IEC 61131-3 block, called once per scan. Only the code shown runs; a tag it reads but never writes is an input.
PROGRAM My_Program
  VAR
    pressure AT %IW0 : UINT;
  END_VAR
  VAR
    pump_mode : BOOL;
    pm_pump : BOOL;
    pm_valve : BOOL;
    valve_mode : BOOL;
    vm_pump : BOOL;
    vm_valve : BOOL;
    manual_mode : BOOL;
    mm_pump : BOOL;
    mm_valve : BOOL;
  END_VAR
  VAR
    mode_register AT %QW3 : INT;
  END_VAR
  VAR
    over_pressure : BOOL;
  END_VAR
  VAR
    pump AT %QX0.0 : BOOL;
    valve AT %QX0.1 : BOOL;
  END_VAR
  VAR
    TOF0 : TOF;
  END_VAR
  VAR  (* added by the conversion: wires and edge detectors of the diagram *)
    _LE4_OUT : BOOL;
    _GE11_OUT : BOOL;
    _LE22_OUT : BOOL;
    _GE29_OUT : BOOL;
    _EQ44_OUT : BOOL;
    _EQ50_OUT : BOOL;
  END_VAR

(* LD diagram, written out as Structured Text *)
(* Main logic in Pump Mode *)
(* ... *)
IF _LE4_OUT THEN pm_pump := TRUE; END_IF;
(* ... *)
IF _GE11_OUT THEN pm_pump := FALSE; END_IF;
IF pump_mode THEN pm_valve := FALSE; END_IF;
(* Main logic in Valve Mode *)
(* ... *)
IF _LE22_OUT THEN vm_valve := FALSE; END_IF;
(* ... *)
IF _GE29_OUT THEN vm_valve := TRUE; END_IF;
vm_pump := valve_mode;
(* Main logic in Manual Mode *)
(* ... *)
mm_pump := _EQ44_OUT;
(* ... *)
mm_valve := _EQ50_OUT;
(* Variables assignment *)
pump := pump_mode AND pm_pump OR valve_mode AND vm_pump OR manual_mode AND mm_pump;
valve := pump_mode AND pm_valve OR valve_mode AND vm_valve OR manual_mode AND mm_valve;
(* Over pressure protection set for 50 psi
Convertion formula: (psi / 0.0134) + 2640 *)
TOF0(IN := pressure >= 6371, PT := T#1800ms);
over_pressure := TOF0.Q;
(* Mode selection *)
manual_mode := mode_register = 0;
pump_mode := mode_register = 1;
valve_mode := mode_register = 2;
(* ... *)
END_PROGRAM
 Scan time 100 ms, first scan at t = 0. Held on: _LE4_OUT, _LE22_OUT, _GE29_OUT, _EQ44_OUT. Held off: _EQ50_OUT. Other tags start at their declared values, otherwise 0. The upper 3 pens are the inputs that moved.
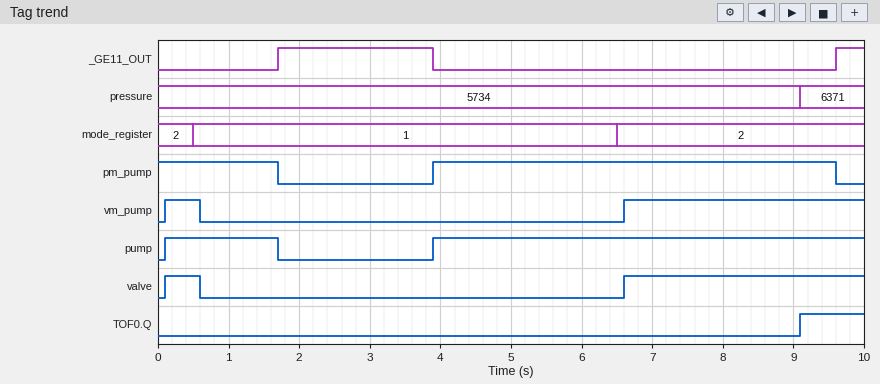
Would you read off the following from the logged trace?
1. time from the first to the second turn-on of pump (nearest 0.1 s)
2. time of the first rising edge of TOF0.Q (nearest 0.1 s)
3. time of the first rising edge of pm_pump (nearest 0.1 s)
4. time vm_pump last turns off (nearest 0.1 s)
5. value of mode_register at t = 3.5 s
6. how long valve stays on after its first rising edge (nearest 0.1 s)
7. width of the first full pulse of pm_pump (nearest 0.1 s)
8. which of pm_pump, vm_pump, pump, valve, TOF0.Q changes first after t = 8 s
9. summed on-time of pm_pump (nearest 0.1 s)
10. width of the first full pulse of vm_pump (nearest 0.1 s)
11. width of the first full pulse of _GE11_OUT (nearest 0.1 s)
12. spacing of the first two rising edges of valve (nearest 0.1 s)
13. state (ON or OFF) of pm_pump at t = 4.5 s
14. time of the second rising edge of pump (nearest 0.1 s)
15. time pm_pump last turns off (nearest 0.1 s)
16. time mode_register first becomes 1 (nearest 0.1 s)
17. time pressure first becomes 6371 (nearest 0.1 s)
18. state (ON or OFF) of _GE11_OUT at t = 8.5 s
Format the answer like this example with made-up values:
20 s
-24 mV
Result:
3.8 s
9.1 s
3.9 s
0.6 s
1
0.5 s
5.7 s
TOF0.Q
7.4 s
0.5 s
2.2 s
6.5 s
ON
3.9 s
9.6 s
0.5 s
9.1 s
OFF
